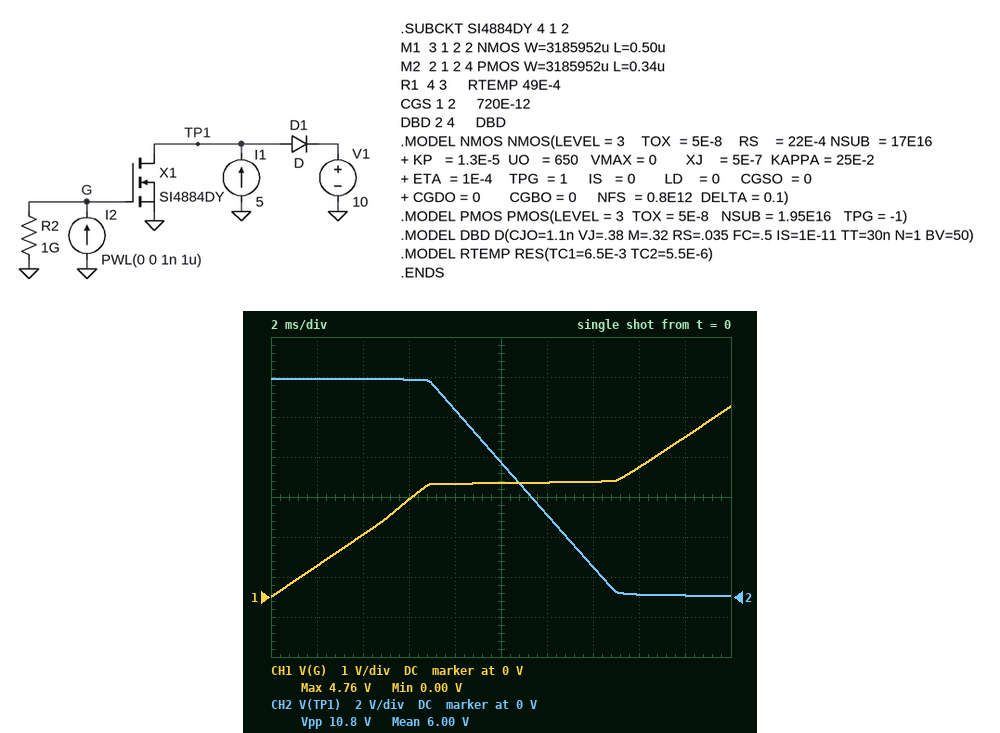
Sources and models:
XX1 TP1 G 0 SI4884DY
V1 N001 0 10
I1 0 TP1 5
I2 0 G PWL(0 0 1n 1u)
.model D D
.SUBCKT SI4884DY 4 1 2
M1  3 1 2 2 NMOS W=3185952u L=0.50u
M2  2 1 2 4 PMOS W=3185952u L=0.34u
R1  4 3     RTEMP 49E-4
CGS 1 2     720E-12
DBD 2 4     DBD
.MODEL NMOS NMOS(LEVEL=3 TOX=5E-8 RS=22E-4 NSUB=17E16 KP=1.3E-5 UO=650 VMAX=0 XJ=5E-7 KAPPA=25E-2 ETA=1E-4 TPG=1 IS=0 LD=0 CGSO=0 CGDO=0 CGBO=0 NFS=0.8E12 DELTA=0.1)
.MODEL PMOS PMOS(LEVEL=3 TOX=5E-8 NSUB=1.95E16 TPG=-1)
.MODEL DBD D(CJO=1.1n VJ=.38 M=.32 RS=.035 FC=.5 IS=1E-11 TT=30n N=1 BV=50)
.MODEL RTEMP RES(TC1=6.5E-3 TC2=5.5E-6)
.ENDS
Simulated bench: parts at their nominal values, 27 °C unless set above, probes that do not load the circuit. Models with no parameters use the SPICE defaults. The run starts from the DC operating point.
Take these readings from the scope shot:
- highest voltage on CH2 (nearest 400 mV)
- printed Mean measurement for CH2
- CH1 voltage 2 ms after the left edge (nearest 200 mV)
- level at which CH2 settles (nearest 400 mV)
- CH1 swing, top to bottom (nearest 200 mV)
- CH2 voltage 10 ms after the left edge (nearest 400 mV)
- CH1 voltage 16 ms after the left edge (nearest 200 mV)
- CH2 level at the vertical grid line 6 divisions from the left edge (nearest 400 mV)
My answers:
10.8 V
6.00 V
800 mV
0 V
4.8 V
6.8 V
3.2 V
4.0 V
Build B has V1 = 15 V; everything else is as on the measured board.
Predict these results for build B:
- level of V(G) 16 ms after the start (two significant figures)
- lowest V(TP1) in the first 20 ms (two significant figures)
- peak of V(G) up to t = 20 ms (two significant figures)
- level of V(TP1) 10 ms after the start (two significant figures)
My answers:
2.9 V
110 mV
3.3 V
12 V
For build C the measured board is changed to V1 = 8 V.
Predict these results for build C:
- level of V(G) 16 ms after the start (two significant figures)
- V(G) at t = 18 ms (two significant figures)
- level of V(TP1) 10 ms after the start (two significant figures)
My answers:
3.8 V
4.6 V
4.8 V
